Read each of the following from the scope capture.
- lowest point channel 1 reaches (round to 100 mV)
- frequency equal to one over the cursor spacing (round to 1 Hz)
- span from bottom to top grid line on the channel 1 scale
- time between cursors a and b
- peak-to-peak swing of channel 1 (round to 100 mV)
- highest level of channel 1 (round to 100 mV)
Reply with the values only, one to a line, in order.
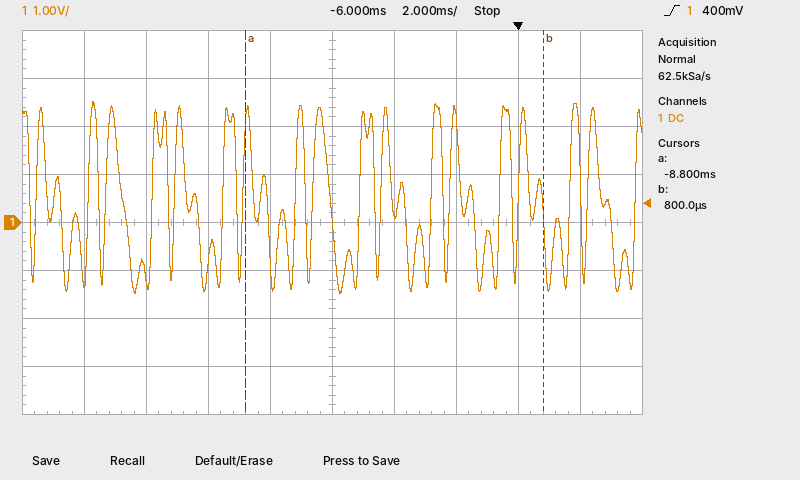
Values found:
-1.5 V
104 Hz
8 V
9.6 ms
4.0 V
2.5 V
